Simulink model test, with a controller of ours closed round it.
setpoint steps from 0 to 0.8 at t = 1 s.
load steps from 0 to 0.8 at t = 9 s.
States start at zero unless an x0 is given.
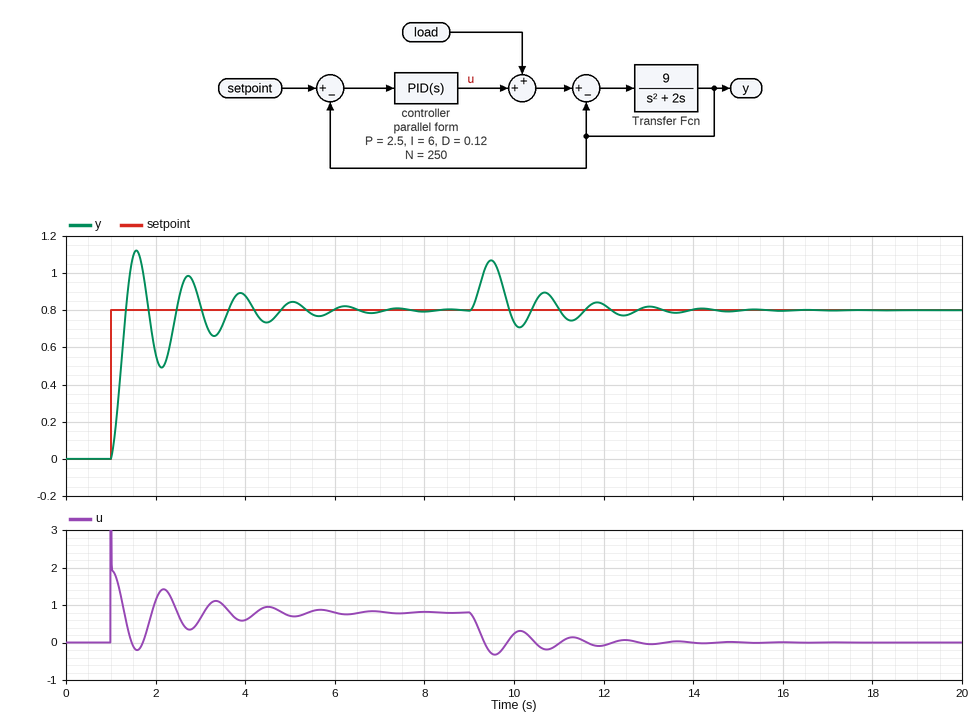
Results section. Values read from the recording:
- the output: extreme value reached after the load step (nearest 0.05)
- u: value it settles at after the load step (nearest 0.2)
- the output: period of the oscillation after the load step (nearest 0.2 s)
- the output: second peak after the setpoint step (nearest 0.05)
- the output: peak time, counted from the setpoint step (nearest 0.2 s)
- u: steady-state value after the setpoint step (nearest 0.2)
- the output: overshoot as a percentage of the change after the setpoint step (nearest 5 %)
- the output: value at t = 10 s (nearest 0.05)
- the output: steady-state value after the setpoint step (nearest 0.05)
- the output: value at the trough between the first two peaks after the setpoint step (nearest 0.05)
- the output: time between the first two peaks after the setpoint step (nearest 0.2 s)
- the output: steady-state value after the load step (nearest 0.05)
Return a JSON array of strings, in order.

["1.05", "0.0", "1.2 s", "1.00", "0.6 s", "0.8", "40 %", "0.75", "0.80", "0.50", "1.2 s", "0.80"]
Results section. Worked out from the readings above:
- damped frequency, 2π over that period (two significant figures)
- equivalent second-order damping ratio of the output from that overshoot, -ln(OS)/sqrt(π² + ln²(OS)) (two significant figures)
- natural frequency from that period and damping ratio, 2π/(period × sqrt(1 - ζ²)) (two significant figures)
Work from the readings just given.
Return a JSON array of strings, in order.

["5.2 rad/s", "0.28", "5.5 rad/s"]
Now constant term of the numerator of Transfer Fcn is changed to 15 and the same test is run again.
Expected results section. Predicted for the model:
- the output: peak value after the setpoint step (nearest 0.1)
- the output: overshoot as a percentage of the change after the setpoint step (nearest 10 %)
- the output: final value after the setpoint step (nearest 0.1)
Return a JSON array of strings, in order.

["1.1", "30 %", "0.8"]
